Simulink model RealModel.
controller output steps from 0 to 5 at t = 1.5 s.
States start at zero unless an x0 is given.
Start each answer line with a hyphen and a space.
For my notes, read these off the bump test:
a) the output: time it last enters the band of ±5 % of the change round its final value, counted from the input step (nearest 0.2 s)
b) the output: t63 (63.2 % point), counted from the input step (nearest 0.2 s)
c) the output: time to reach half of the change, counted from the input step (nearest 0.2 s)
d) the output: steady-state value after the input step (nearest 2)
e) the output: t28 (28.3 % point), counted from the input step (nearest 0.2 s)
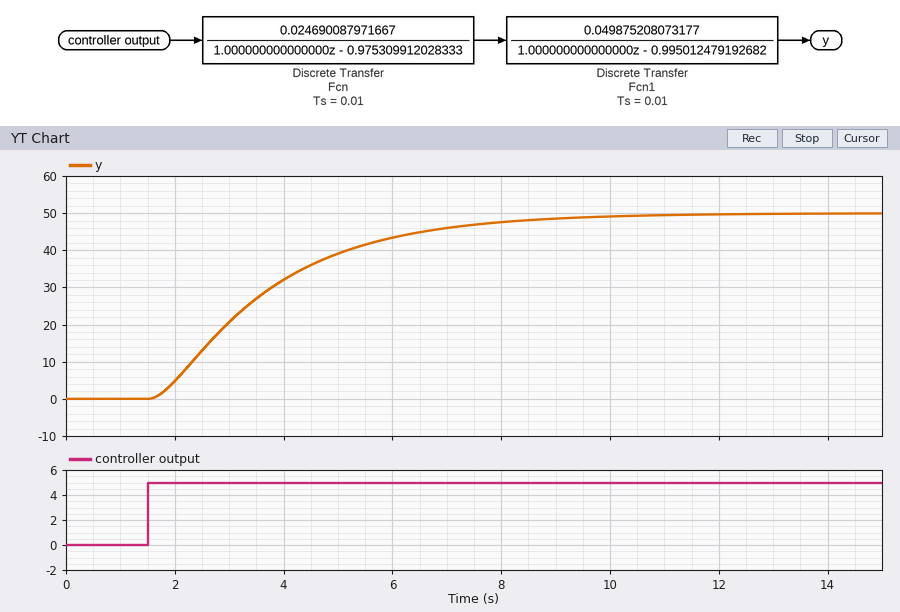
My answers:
- 6.4 s
- 2.4 s
- 1.8 s
- 50
- 1.0 s
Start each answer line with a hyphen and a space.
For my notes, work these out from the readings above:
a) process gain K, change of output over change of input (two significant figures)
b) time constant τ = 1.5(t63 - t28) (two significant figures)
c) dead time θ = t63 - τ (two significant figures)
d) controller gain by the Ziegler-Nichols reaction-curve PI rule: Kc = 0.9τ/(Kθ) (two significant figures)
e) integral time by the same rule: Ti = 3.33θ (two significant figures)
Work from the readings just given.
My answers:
- 10
- 2.1 s
- 0.30 s
- 0.63
- 1.00 s
